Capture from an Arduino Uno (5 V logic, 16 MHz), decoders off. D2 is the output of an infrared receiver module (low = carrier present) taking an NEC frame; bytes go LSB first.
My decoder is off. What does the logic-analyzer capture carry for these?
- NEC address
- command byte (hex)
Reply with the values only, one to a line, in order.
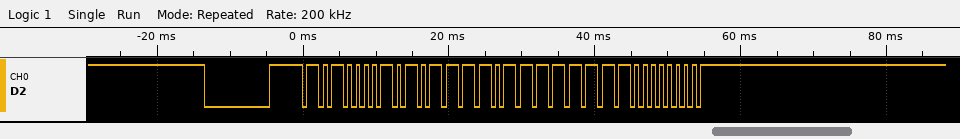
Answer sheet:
0x85
0xFF
